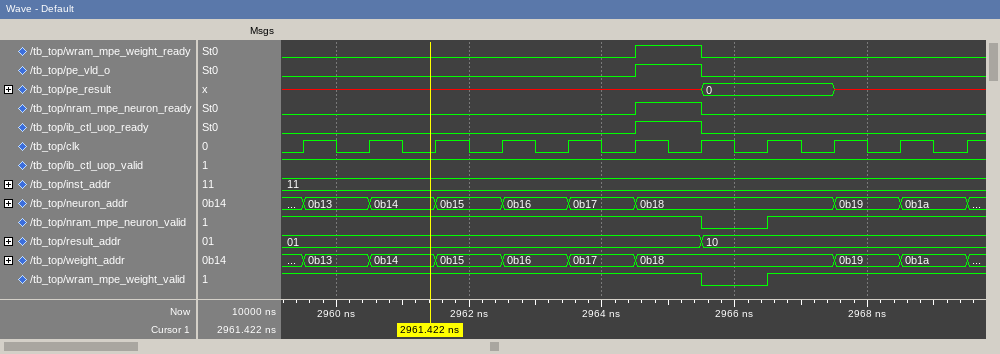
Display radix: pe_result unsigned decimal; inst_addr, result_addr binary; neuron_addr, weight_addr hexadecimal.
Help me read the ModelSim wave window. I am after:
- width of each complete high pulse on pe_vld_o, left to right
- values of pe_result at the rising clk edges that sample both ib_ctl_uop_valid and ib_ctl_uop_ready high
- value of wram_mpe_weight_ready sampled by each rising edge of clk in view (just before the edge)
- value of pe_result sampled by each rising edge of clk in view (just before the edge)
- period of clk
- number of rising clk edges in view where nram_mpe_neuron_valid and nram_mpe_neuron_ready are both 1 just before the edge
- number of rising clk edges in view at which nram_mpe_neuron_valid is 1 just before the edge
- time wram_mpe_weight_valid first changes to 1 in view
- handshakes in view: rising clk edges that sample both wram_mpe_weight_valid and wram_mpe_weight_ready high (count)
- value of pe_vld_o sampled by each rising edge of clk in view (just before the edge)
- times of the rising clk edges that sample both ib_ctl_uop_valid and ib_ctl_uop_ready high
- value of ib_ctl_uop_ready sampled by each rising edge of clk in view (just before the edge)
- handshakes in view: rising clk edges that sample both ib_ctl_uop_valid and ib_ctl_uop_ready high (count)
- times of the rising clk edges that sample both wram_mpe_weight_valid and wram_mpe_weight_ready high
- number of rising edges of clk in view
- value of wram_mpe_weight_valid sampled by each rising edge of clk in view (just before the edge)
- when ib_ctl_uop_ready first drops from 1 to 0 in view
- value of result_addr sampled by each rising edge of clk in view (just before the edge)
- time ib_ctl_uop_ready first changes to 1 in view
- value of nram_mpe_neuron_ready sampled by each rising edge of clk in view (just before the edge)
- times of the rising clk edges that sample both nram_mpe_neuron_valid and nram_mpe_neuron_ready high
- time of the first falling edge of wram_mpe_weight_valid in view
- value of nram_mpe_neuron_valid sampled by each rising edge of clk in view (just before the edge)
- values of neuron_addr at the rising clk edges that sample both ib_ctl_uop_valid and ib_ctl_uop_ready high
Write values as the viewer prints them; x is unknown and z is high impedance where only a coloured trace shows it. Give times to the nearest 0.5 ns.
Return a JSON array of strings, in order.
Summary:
["1 ns", "x", "0 0 0 0 0 0 1 0 0 0 0", "x, x, x, x, x, x, x, 0, 0, x, x", "1 ns", "1", "10", "2966.5 ns", "1", "0 0 0 0 0 0 1 0 0 0 0", "2965.5 ns", "0 0 0 0 0 0 1 0 0 0 0", "1", "2965.5 ns", "11", "1 1 1 1 1 1 1 0 1 1 1", "2965.5 ns", "01, 01, 01, 01, 01, 01, 01, 10, 10, 10, 10", "2964.5 ns", "0 0 0 0 0 0 1 0 0 0 0", "2965.5 ns", "2965.5 ns", "1 1 1 1 1 1 1 0 1 1 1", "0b18"]
